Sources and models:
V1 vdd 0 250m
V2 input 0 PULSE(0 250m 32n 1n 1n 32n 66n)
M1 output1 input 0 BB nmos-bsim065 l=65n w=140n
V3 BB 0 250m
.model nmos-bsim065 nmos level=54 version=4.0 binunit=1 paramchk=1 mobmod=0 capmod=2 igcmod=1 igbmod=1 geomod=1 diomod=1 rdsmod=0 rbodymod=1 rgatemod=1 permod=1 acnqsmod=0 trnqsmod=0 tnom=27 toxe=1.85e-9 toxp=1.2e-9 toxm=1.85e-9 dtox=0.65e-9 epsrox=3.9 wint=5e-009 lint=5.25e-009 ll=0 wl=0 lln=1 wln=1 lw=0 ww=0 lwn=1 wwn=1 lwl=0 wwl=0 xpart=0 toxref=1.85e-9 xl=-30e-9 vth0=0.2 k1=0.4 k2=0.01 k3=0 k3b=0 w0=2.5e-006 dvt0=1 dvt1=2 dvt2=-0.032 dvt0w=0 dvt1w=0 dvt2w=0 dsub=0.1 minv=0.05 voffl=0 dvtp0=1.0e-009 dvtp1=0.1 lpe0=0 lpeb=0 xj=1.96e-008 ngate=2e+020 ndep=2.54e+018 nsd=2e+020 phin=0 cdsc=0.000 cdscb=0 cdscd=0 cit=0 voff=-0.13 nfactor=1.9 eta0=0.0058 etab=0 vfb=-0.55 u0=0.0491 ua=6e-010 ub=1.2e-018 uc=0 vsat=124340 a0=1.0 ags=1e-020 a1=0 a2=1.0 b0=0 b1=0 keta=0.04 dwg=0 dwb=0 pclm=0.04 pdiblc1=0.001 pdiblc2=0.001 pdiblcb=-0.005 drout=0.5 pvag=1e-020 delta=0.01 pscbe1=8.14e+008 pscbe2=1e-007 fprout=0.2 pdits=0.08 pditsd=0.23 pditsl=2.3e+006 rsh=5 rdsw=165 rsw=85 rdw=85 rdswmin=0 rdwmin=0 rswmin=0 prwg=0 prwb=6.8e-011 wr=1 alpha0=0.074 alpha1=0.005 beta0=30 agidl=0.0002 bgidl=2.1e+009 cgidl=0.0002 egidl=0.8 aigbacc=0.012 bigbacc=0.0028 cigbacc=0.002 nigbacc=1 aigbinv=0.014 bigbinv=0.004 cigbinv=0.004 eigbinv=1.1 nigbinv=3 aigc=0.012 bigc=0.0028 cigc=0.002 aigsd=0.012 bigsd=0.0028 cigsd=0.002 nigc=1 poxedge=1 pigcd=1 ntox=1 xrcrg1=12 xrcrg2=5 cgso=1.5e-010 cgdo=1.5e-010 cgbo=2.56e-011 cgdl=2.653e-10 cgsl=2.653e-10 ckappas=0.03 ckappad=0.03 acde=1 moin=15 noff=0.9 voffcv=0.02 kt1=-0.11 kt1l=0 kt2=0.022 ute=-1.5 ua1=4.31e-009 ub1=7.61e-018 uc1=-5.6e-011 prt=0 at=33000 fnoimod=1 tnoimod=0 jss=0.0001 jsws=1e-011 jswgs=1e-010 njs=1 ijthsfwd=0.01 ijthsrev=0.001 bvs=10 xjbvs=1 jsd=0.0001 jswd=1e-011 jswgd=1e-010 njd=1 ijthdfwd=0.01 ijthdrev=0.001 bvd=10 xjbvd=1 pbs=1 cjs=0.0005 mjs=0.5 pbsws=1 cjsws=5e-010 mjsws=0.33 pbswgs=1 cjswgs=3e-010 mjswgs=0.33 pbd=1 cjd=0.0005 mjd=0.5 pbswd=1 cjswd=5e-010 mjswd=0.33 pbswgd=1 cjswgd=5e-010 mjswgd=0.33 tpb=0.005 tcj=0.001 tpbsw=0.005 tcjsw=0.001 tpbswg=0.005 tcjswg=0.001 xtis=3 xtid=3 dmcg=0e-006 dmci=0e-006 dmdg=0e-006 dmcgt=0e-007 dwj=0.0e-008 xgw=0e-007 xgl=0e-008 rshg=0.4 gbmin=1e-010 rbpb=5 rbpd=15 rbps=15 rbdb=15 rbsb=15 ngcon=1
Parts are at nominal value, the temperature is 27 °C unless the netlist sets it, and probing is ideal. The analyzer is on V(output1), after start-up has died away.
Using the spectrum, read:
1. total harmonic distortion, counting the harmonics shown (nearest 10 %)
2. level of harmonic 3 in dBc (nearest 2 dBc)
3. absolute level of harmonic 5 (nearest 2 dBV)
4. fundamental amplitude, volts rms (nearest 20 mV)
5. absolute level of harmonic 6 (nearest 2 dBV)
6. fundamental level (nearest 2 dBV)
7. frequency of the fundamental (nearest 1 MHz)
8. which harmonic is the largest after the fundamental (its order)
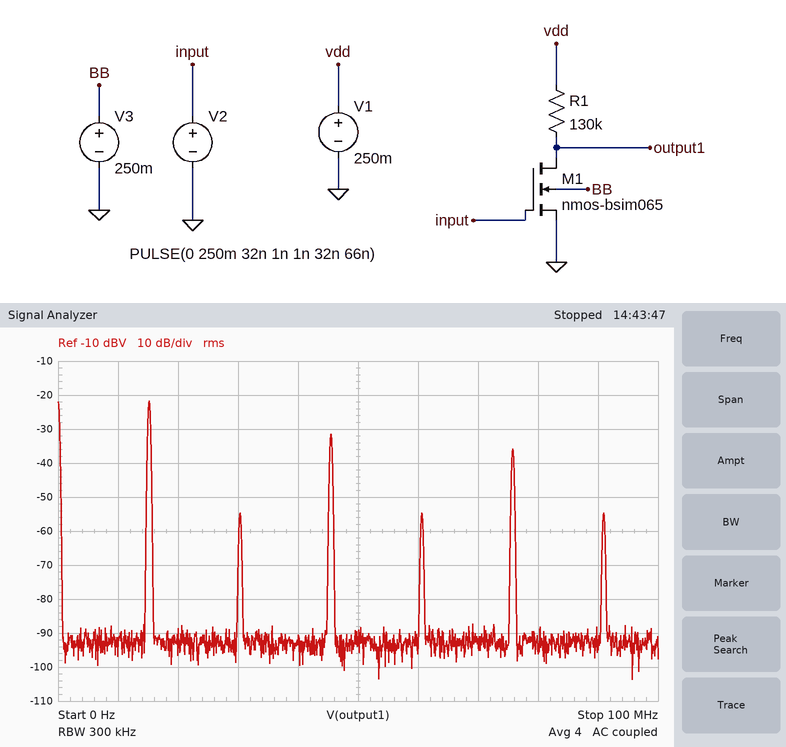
40 %
-10 dBc
-36 dBV
80 mV
-54 dBV
-22 dBV
15 MHz
3
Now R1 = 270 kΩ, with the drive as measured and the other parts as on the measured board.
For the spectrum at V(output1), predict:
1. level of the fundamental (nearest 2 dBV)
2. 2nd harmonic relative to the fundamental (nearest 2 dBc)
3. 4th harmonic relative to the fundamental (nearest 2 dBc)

-24 dBV
-30 dBc
-30 dBc
